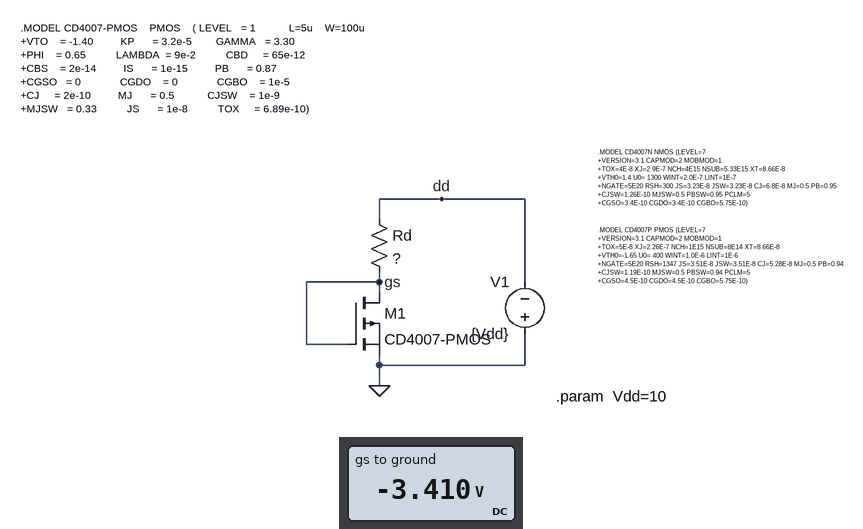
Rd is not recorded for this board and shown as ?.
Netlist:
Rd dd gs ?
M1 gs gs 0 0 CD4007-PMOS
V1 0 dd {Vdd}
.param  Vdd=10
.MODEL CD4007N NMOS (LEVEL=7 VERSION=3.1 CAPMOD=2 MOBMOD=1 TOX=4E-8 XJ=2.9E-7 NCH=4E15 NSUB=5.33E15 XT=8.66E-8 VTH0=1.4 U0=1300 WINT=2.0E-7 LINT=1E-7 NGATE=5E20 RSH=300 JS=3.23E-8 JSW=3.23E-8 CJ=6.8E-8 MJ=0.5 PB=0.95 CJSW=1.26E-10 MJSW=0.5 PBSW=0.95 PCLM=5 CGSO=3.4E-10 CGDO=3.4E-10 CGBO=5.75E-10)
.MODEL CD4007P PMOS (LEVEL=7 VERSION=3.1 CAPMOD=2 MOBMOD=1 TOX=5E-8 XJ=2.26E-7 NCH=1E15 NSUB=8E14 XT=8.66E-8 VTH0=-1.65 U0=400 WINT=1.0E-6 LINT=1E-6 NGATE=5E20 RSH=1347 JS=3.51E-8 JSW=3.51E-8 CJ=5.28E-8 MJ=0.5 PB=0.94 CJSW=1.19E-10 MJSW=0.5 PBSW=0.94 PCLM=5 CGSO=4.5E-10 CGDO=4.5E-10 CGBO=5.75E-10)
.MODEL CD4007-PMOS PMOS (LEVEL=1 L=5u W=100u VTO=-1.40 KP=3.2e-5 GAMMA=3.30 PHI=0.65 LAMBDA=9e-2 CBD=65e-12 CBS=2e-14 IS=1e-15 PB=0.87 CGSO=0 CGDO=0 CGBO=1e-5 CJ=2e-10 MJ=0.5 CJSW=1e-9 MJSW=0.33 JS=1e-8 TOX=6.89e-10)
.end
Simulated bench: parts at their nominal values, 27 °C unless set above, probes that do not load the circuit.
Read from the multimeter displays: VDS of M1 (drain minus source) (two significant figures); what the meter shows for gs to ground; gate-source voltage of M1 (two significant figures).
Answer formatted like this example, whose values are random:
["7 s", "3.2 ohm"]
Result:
["-3.4 V", "-3.410 V", "-3.4 V"]
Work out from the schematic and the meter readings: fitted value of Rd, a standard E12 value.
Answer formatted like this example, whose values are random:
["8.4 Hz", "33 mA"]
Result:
["3.9 kΩ"]
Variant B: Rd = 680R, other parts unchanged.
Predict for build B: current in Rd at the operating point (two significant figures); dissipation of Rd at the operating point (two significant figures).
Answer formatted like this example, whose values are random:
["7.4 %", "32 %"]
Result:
["7.0 mA", "33 mW"]
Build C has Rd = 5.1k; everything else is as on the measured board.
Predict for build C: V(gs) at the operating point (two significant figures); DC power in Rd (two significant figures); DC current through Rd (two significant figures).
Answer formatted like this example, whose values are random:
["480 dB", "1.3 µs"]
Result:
["-3.2 V", "9.1 mW", "1.3 mA"]
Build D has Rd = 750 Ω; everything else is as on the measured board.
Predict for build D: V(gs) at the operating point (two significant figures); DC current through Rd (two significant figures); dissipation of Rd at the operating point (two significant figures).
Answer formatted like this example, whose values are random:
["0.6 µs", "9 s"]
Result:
["-5.1 V", "6.5 mA", "32 mW"]
